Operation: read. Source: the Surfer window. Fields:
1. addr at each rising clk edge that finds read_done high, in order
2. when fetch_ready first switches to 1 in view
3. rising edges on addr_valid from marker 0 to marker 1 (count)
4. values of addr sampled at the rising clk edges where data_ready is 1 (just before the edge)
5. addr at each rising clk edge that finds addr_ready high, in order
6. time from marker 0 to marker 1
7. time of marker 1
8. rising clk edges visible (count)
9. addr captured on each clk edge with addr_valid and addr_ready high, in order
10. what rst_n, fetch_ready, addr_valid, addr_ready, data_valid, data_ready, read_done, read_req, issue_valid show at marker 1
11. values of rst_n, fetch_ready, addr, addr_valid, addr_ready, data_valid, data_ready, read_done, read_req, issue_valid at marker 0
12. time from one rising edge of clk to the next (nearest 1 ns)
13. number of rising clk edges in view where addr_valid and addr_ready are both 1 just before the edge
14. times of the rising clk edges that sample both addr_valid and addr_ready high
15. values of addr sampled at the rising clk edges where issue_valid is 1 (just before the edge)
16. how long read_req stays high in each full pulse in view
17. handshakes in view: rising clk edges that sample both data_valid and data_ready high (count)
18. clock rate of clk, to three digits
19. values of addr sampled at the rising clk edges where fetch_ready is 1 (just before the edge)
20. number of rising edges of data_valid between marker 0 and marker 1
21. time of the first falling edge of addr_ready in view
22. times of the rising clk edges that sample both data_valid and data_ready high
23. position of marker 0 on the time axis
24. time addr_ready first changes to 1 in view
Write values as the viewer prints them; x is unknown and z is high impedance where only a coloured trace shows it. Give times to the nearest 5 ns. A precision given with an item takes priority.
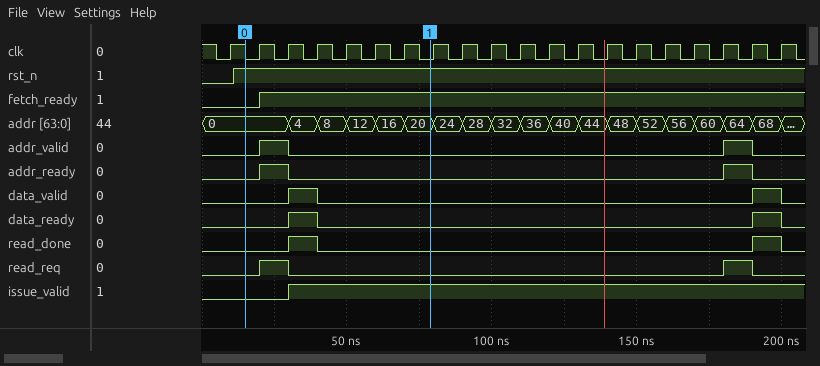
4, 68
20 ns
1
4, 68
0, 64
65 ns
80 ns
20
0, 64
rst_n=1, fetch_ready=1, addr_valid=0, addr_ready=0, data_valid=0, data_ready=0, read_done=0, read_req=0, issue_valid=1
rst_n=1, fetch_ready=0, addr=0, addr_valid=0, addr_ready=0, data_valid=0, data_ready=0, read_done=0, read_req=0, issue_valid=0
10 ns
2
30 ns, 190 ns
4, 8, 12, 16, 20, 24, 28, 32, 36, 40, 44, 48, 52, 56, 60, 64, 68
10 ns, 10 ns
2
100 MHz
0, 4, 8, 12, 16, 20, 24, 28, 32, 36, 40, 44, 48, 52, 56, 60, 64, 68
1
30 ns
40 ns, 200 ns
15 ns
20 ns
